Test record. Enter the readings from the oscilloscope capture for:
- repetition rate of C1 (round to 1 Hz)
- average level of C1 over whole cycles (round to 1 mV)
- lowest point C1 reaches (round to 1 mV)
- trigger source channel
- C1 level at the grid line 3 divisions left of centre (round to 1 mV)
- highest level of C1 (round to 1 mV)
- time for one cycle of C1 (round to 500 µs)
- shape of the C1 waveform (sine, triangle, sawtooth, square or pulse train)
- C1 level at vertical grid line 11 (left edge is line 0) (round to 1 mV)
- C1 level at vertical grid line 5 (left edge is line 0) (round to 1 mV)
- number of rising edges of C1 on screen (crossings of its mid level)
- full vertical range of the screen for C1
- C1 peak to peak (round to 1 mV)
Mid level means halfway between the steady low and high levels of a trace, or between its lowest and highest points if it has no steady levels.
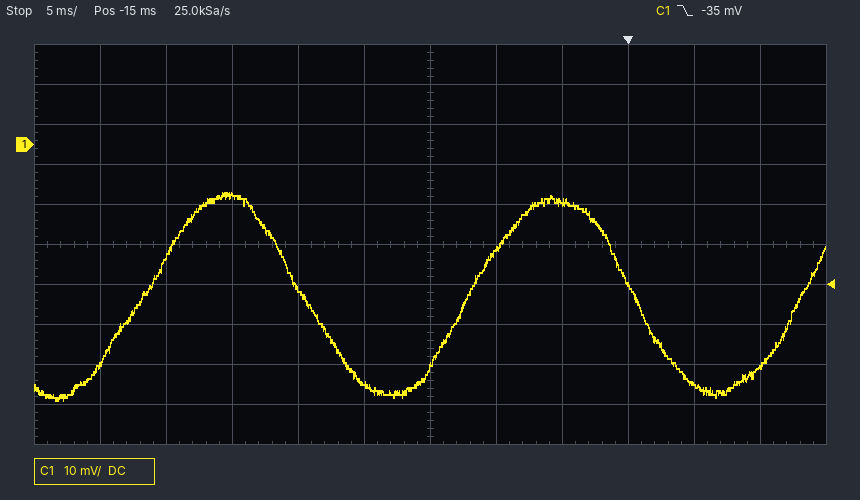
40 Hz
-38 mV
-64 mV
C1
-13 mV
-12 mV
25.0 ms
sine
-55 mV
-60 mV
3
100 mV
52 mV
